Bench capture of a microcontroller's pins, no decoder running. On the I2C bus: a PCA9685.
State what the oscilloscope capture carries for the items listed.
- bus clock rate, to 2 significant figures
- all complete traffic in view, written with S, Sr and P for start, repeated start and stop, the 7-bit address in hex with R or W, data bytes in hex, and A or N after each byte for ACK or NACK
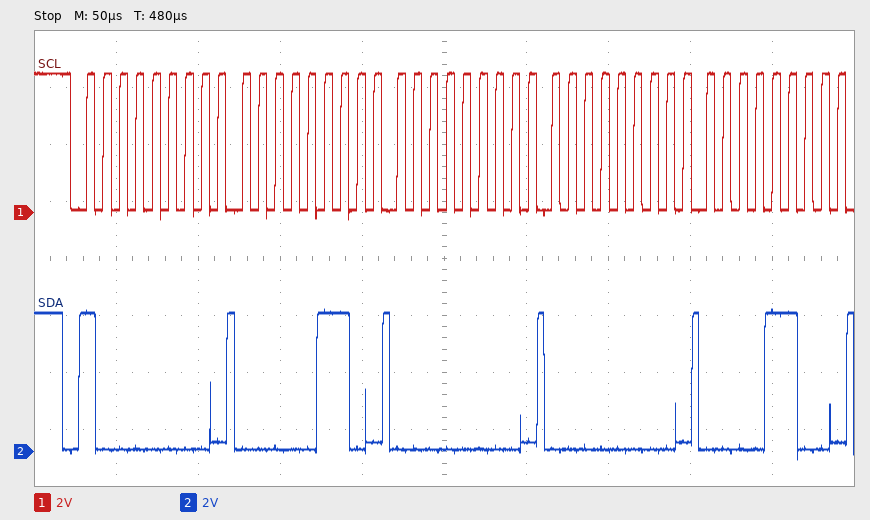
100 kHz
S 40W A 06 A 00 A 00 A 0C A
